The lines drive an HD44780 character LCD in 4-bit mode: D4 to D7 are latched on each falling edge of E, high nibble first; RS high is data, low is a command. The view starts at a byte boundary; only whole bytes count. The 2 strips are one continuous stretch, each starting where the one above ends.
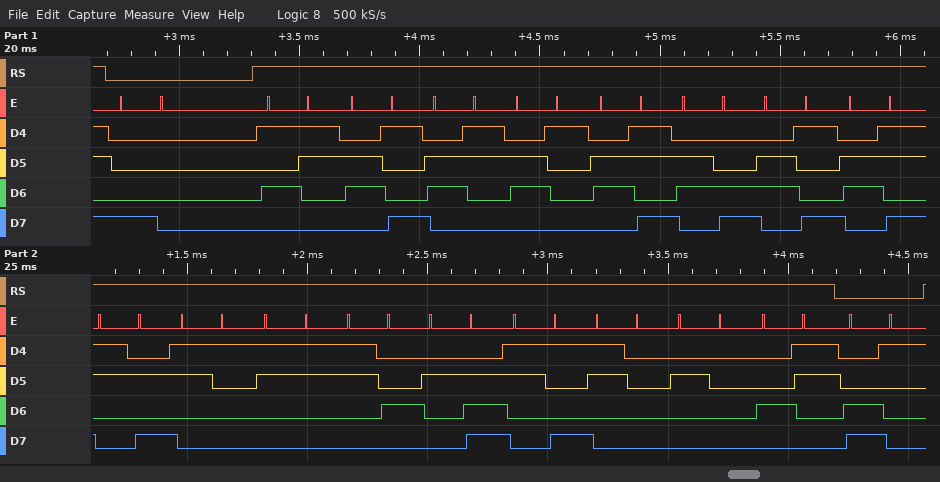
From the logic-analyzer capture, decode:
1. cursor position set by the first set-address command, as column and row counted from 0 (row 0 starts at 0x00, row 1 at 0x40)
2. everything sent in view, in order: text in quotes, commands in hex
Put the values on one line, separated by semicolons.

column 0, row 0; 0x80 "Sicaklik:134.90 C" 0xC1
